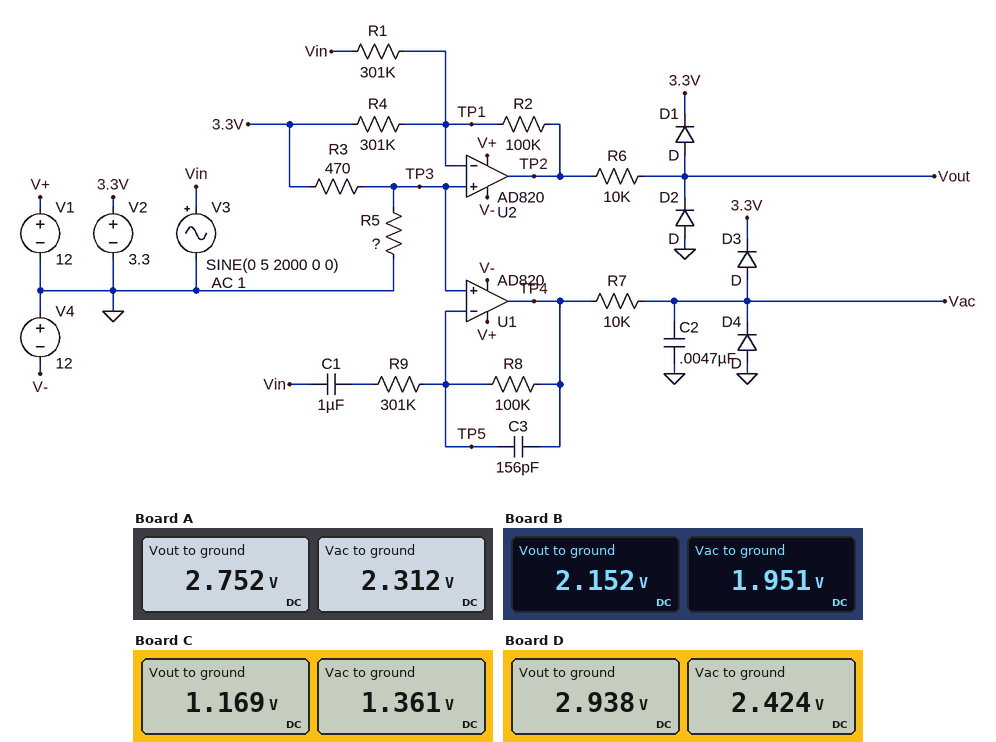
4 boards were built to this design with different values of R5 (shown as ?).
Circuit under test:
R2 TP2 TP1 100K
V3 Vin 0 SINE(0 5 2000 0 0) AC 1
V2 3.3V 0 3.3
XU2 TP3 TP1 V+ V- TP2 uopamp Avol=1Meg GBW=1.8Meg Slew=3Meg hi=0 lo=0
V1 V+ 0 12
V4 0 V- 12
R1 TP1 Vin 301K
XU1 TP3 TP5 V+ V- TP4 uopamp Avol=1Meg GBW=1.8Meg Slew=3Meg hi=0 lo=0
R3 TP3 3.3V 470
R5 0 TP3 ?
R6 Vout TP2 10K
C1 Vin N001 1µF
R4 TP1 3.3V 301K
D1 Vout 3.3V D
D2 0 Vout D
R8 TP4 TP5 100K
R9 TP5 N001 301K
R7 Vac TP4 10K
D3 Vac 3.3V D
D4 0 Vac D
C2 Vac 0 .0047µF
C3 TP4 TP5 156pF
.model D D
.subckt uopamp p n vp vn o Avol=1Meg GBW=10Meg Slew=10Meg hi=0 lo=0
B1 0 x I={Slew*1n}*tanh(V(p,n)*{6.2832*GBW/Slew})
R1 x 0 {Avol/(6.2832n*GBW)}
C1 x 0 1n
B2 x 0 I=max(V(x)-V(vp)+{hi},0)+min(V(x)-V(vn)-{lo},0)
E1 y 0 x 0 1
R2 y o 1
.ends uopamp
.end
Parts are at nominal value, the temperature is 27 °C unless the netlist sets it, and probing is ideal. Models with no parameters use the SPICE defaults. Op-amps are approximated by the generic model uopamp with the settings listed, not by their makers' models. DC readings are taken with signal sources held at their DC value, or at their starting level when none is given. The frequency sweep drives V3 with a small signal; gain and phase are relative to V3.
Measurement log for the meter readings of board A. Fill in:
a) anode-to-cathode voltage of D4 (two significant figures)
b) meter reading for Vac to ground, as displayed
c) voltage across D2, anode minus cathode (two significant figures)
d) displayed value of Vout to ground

-2.3 V
2.312 V
-2.8 V
2.752 V
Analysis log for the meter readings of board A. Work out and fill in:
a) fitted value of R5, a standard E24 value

1.1 kΩ
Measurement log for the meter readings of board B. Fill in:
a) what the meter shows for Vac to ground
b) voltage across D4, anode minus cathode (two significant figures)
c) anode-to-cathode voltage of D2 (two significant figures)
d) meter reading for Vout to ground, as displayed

1.951 V
-2.0 V
-2.2 V
2.152 V
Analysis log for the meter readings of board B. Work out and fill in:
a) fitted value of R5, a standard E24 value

680 Ω
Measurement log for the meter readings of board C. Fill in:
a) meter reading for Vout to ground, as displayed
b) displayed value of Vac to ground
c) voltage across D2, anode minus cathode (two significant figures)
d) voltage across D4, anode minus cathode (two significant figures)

1.169 V
1.361 V
-1.2 V
-1.4 V
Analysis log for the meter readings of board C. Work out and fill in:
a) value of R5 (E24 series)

330 Ω
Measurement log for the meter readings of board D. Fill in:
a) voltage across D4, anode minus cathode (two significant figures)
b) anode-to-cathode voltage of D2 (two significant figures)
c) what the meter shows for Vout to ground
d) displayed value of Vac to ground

-2.4 V
-2.9 V
2.938 V
2.424 V
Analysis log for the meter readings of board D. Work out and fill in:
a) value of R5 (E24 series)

1.3 kΩ
